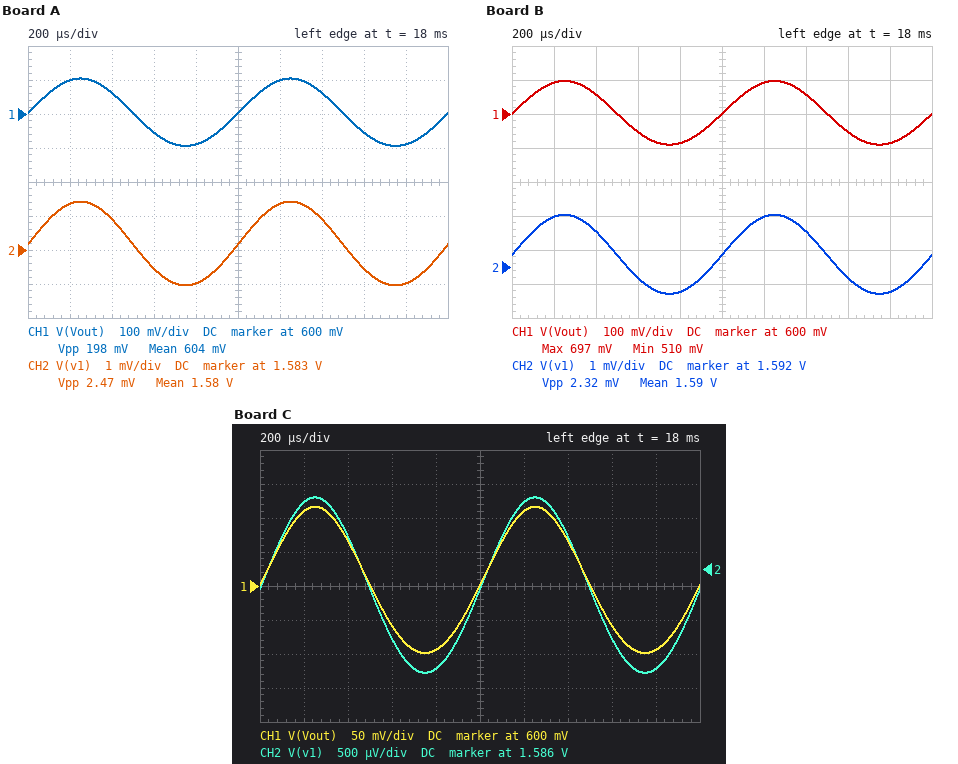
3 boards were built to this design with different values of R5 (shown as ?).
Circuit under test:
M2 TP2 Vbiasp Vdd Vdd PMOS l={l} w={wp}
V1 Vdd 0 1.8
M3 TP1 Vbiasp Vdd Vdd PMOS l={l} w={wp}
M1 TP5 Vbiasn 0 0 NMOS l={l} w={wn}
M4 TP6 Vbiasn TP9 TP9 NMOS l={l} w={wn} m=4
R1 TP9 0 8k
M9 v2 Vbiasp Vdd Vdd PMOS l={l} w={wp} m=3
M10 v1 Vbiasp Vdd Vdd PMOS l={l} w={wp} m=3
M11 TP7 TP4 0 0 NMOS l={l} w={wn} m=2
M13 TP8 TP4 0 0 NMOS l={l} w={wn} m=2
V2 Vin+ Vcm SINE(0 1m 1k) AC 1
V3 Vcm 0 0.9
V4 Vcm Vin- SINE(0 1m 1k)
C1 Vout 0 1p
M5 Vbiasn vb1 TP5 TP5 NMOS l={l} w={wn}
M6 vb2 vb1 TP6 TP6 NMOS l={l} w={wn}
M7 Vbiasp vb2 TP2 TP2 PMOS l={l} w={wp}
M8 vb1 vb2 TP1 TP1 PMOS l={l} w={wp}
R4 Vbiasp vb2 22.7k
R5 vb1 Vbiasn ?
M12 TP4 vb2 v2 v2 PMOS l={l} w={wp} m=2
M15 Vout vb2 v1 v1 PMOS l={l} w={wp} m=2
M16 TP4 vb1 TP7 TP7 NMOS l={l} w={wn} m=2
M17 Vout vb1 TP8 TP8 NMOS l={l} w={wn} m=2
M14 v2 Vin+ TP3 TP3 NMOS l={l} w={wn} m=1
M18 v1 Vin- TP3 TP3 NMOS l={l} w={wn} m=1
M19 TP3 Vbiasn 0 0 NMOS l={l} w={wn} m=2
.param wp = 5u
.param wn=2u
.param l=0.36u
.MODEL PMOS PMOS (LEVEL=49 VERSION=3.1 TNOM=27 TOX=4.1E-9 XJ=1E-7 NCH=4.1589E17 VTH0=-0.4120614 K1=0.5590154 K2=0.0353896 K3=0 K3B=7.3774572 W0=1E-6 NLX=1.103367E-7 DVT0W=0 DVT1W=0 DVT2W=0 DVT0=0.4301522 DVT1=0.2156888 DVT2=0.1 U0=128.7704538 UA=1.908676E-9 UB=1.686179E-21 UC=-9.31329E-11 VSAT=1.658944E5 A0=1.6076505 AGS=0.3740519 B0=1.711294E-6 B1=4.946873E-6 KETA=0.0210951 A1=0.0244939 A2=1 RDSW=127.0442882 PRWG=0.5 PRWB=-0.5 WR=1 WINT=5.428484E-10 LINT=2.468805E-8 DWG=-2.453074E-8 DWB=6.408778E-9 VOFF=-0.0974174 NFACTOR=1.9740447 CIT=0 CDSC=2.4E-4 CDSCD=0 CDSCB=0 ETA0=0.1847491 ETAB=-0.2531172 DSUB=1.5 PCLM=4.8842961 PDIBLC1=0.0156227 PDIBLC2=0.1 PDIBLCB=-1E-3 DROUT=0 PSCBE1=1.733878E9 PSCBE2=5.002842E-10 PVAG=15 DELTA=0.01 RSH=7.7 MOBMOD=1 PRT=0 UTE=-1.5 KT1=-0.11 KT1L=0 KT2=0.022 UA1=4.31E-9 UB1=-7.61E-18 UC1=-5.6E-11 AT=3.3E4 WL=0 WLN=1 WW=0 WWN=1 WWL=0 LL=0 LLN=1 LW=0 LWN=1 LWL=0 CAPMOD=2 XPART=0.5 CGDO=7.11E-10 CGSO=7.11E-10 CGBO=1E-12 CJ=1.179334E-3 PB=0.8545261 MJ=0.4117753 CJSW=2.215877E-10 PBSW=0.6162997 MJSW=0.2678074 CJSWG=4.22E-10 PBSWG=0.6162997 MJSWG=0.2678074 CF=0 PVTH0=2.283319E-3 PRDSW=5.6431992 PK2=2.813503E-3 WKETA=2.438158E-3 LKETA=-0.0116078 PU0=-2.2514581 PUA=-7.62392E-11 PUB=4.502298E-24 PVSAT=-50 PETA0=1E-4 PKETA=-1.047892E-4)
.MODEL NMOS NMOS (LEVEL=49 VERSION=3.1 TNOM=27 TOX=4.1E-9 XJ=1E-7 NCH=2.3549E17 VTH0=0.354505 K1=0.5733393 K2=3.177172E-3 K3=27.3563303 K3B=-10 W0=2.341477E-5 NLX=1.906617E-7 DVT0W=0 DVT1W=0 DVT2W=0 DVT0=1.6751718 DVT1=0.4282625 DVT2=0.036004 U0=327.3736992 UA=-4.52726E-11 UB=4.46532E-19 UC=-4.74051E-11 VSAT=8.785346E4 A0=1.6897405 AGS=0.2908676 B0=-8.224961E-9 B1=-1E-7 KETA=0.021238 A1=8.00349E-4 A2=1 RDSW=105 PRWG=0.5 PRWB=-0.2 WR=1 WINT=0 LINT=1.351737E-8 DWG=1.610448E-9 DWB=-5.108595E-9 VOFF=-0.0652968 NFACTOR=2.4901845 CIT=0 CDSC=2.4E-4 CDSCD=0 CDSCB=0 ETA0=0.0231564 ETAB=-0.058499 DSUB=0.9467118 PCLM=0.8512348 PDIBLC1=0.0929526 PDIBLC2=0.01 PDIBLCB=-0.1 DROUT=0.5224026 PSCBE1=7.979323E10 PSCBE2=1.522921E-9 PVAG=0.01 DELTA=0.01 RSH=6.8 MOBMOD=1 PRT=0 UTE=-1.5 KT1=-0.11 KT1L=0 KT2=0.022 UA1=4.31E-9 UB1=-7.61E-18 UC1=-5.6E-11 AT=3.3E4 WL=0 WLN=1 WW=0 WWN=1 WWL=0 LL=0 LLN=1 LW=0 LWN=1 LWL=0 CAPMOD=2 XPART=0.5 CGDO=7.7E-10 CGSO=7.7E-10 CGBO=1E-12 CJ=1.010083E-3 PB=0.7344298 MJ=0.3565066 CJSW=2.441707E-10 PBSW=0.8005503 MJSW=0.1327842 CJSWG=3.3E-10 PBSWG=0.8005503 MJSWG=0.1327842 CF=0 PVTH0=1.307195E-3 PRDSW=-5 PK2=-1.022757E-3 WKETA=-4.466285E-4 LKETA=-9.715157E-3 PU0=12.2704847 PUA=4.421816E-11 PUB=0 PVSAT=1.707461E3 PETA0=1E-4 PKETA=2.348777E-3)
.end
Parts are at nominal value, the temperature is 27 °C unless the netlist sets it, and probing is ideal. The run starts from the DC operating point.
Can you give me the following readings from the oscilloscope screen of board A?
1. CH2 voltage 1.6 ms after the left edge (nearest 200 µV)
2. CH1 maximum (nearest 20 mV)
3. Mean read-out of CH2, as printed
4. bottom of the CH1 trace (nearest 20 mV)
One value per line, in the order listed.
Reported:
1.5824 V
700 mV
1.58 V
500 mV
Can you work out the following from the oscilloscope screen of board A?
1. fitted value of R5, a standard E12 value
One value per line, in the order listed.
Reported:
100 kΩ
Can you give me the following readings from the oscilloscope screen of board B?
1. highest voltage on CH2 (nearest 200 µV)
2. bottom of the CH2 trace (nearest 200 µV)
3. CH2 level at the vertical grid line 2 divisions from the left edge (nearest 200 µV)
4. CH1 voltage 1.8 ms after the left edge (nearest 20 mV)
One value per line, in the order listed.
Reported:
1.5936 V
1.5912 V
1.5930 V
520 mV
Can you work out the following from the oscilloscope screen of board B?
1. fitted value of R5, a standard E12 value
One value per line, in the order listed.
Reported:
120 kΩ
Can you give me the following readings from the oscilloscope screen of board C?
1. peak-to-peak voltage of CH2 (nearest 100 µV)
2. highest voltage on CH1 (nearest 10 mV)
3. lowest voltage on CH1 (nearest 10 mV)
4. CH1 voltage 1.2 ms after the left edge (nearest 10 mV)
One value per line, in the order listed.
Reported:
2.6 mV
720 mV
500 mV
710 mV
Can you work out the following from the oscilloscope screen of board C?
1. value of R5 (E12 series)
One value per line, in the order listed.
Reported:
82 kΩ
